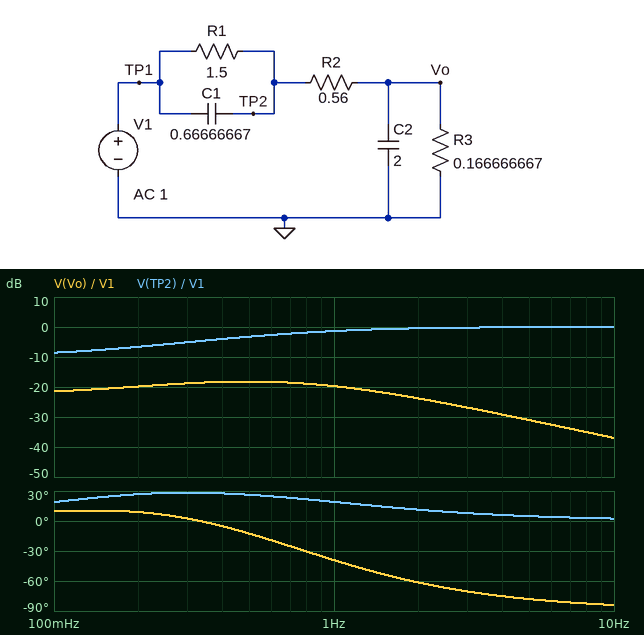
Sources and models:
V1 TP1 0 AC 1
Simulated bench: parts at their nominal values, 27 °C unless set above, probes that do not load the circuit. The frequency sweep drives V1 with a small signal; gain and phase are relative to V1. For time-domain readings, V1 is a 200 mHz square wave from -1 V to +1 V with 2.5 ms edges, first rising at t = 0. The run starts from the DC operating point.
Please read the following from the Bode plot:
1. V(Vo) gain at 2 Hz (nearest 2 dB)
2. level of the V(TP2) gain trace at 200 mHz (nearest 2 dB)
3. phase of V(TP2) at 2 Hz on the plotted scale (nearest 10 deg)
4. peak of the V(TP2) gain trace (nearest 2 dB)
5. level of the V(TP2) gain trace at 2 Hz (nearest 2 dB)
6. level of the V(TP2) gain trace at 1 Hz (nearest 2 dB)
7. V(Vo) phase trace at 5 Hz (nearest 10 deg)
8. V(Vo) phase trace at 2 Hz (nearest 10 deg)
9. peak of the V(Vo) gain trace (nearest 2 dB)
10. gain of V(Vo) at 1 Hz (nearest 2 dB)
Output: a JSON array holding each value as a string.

["-24 dB", "-6 dB", "10 deg", "0 dB", "0 dB", "-2 dB", "-80 deg", "-60 deg", "-18 dB", "-20 dB"]
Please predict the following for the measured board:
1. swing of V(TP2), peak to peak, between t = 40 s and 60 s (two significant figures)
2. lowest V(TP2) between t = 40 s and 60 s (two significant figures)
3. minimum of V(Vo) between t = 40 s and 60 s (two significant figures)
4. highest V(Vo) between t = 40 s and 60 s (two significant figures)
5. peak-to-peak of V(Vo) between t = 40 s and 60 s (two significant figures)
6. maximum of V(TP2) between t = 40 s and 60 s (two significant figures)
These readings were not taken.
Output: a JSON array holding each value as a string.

["3.3 V", "-1.7 V", "-150 mV", "150 mV", "300 mV", "1.7 V"]
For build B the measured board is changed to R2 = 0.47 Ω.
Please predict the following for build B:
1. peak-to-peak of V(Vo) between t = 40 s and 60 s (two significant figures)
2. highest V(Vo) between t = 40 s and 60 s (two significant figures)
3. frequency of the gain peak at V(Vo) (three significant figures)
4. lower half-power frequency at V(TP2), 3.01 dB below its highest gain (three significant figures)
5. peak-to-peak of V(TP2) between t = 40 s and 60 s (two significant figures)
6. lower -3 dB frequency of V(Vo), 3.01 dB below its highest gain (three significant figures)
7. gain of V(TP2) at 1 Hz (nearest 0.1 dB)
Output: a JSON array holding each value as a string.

["330 mV", "160 mV", "530 mHz", "629 mHz", "3.4 V", "134 mHz", "-1.7 dB"]
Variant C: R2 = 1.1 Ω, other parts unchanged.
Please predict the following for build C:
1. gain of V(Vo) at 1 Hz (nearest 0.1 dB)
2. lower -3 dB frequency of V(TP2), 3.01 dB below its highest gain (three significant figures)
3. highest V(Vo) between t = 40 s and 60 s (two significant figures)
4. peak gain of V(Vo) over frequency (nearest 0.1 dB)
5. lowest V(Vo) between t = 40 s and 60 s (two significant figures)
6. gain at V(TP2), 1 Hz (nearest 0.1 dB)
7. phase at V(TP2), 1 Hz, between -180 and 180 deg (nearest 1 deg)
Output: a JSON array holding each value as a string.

["-24.5 dB", "285 mHz", "97 mV", "-21.5 dB", "-97 mV", "-0.5 dB", "11 deg"]
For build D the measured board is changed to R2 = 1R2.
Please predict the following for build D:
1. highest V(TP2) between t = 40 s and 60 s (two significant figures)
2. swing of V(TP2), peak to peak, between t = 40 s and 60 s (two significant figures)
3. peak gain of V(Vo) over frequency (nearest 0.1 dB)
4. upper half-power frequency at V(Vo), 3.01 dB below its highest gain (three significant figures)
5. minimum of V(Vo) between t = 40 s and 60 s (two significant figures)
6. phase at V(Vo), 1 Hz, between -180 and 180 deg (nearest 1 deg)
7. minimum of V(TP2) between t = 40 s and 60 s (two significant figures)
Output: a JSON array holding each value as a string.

["1.5 V", "3.0 V", "-22.0 dB", "973 mHz", "-91 mV", "-51 deg", "-1.5 V"]
